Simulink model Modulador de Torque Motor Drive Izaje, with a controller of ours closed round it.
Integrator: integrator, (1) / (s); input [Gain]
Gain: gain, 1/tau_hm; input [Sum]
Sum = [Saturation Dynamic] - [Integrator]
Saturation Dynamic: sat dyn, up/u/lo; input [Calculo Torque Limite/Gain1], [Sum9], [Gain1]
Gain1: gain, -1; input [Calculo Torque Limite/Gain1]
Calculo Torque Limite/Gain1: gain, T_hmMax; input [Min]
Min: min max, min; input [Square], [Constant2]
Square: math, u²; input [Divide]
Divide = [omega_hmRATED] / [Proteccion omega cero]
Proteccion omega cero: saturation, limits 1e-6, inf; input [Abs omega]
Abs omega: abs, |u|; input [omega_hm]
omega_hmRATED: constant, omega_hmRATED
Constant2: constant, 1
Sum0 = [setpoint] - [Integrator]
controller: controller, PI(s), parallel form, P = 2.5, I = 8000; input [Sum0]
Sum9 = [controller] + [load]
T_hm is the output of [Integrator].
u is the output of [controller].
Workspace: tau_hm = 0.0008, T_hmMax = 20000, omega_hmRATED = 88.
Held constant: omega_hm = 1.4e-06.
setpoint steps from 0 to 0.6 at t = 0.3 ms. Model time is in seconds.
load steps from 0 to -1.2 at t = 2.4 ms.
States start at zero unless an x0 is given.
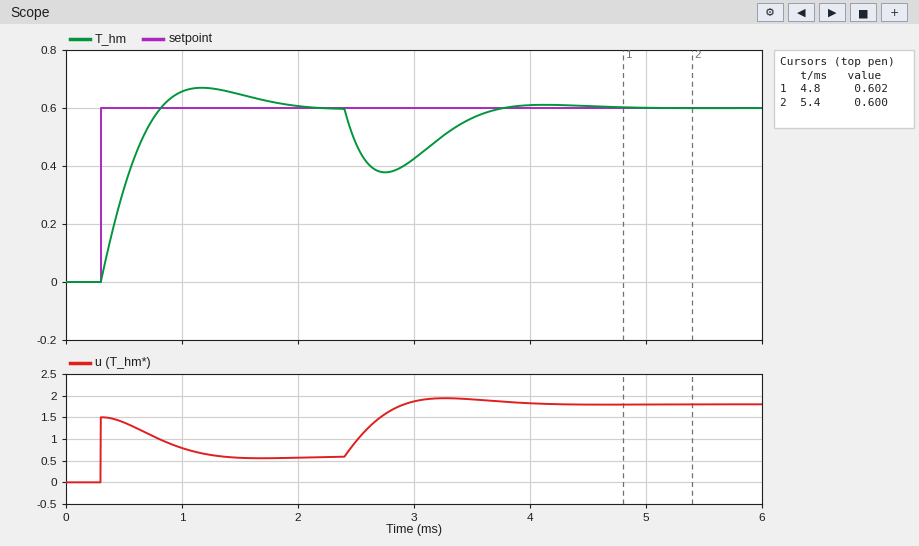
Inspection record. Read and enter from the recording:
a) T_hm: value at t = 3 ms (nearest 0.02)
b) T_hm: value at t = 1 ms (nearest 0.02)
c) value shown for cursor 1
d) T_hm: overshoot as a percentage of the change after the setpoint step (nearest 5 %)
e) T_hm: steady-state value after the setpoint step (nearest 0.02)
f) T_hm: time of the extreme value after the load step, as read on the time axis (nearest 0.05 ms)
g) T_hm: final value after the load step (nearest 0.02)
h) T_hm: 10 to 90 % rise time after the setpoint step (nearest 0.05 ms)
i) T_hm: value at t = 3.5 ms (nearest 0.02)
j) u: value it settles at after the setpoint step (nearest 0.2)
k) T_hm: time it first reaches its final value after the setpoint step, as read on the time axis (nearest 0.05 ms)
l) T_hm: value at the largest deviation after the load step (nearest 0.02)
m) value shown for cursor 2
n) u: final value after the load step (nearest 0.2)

0.42
0.66
0.602
10 %
0.60
2.75 ms
0.60
0.40 ms
0.56
0.6
0.80 ms
0.38
0.600
1.8
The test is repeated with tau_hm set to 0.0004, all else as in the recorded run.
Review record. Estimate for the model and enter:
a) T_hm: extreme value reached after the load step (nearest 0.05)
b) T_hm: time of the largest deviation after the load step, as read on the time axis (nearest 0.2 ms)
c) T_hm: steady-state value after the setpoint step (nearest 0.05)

0.35
2.6 ms
0.60
